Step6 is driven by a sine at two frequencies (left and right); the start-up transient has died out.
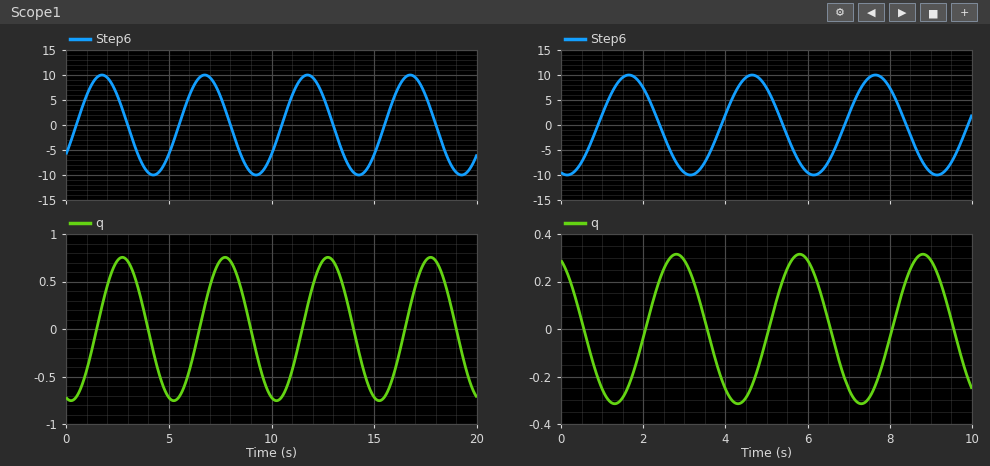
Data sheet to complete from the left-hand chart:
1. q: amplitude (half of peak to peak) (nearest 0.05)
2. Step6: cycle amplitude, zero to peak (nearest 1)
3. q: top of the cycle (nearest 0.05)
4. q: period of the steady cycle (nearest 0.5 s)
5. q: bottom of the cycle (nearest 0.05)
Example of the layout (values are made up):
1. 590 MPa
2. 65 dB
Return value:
1. 0.75
2. 10
3. 0.75
4. 5.0 s
5. -0.75
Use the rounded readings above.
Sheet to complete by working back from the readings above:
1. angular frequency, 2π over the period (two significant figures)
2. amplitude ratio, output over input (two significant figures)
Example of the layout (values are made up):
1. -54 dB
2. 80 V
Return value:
1. 1.3 rad/s
2. 0.075
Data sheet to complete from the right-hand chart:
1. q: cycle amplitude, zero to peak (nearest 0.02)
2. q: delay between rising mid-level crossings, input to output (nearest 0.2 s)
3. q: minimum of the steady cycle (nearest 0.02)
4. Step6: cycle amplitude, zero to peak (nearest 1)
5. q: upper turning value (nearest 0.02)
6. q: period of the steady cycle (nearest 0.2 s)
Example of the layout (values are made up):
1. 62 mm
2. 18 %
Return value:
1. 0.32
2. 1.2 s
3. -0.32
4. 10
5. 0.32
6. 3.0 s
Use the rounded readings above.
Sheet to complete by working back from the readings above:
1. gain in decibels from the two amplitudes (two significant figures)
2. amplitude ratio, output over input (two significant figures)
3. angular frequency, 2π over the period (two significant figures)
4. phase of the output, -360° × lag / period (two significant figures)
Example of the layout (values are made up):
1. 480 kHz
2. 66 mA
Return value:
1. -30 dB
2. 0.032
3. 2.1 rad/s
4. -140°
